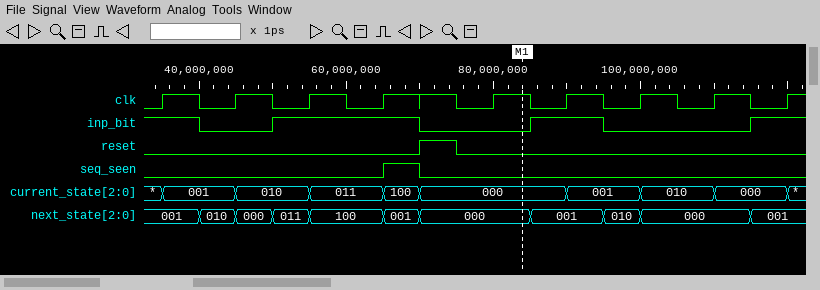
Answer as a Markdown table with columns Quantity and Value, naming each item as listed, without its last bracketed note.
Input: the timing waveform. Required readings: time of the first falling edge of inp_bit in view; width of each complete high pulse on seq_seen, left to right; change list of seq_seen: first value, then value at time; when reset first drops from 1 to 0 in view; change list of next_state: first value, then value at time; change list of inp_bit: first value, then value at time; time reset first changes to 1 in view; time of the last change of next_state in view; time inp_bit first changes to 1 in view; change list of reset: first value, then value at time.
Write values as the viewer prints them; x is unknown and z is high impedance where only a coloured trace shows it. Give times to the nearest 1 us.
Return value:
| Quantity | Value |
|---|---|
| time of the first falling edge of inp_bit in view | 40 us |
| width of each complete high pulse on seq_seen, left to right | 5 us |
| change list of seq_seen: first value, then value at time | 0, 1 at 65 us, 0 at 70 us |
| when reset first drops from 1 to 0 in view | 75 us |
| change list of next_state: first value, then value at time | 001, 010 at 40 us, 000 at 45 us, 011 at 50 us, 100 at 55 us, 001 at 65 us, 000 at 70 us, 001 at 85 us, 010 at 95 us, 000 at 100 us, 001 at 115 us |
| change list of inp_bit: first value, then value at time | 1, 0 at 40 us, 1 at 50 us, 0 at 70 us, 1 at 85 us, 0 at 95 us, 1 at 115 us |
| time reset first changes to 1 in view | 70 us |
| time of the last change of next_state in view | 115 us |
| time inp_bit first changes to 1 in view | 50 us |
| change list of reset: first value, then value at time | 0, 1 at 70 us, 0 at 75 us |
